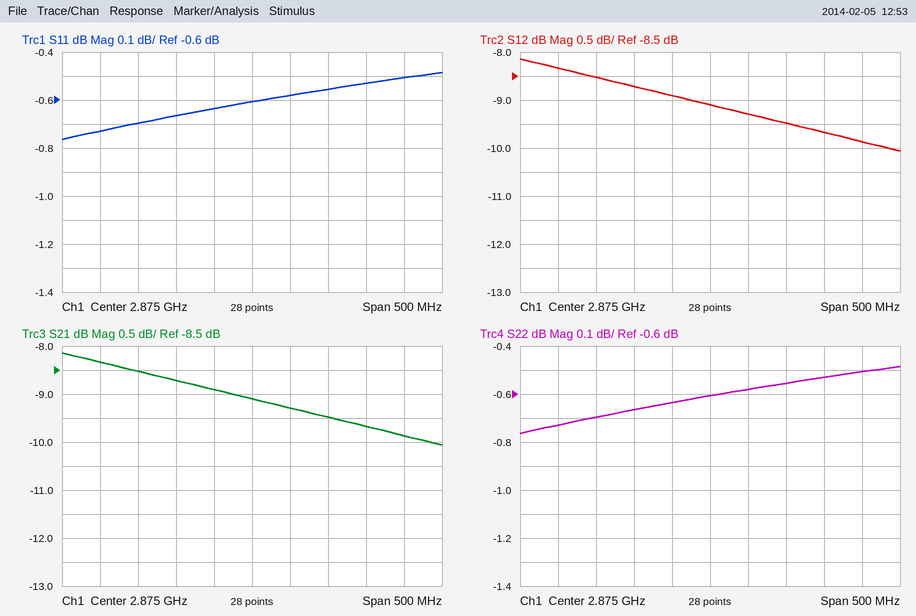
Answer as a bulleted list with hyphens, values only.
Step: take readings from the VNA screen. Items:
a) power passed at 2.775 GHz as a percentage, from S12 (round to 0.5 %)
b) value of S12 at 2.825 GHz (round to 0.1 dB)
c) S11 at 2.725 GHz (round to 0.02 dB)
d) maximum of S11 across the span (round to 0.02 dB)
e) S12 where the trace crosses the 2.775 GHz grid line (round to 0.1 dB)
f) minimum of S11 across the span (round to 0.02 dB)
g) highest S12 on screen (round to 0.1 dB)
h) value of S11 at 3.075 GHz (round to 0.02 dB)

- 13.5 %
- -8.9 dB
- -0.70 dB
- -0.48 dB
- -8.7 dB
- -0.76 dB
- -8.1 dB
- -0.50 dB
